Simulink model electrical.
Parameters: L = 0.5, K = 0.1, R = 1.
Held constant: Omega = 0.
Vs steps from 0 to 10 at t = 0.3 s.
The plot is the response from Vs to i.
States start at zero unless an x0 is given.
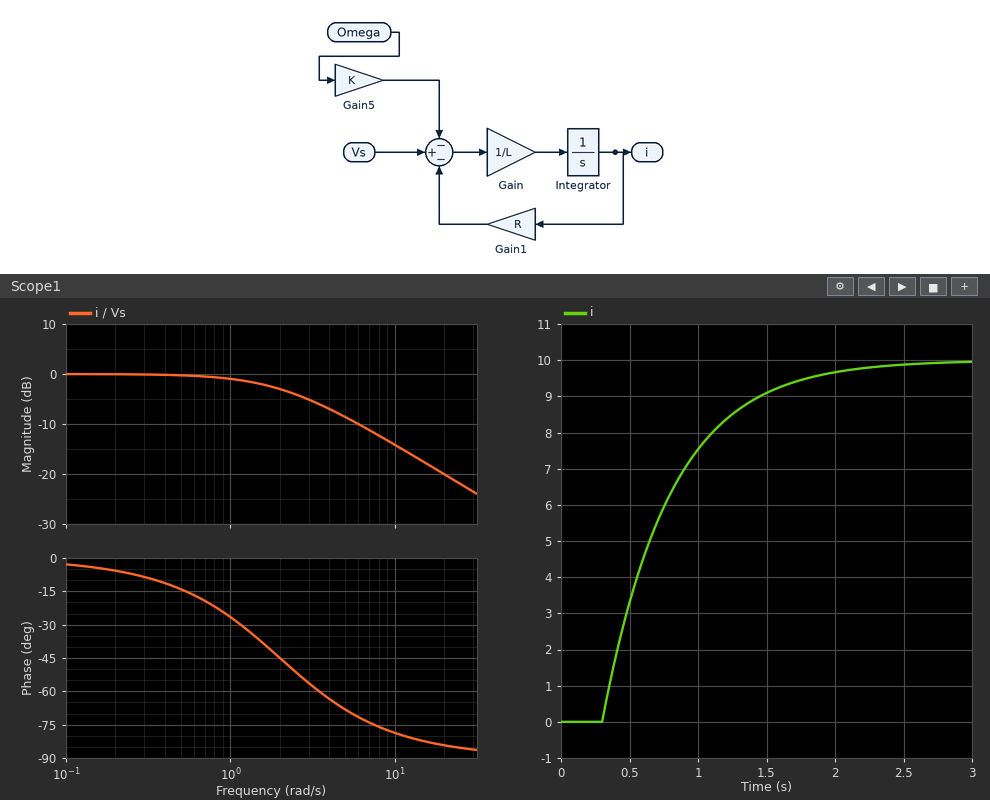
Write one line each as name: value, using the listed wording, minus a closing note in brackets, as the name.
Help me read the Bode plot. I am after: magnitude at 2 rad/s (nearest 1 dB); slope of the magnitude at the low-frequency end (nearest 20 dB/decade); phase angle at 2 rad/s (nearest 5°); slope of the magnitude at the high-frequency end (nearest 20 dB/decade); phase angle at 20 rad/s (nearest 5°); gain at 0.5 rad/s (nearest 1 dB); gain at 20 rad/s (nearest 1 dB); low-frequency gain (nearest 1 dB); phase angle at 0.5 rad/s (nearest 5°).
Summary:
magnitude at 2 rad/s: -3 dB
slope of the magnitude at the low-frequency end: 0 dB/decade
phase angle at 2 rad/s: -45°
slope of the magnitude at the high-frequency end: -20 dB/decade
phase angle at 20 rad/s: -85°
gain at 0.5 rad/s: 0 dB
gain at 20 rad/s: -20 dB
low-frequency gain: 0 dB
phase angle at 0.5 rad/s: -15°
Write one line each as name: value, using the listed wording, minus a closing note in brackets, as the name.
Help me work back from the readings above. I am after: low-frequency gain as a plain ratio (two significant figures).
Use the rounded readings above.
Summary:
low-frequency gain as a plain ratio: 1.0
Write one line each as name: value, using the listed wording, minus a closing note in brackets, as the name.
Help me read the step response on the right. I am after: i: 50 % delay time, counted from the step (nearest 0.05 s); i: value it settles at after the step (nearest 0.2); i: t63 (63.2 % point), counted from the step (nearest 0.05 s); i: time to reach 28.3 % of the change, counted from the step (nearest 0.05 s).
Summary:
i: 50 % delay time, counted from the step: 0.35 s
i: value it settles at after the step: 10.0
i: t63 (63.2 % point), counted from the step: 0.50 s
i: time to reach 28.3 % of the change, counted from the step: 0.15 s
